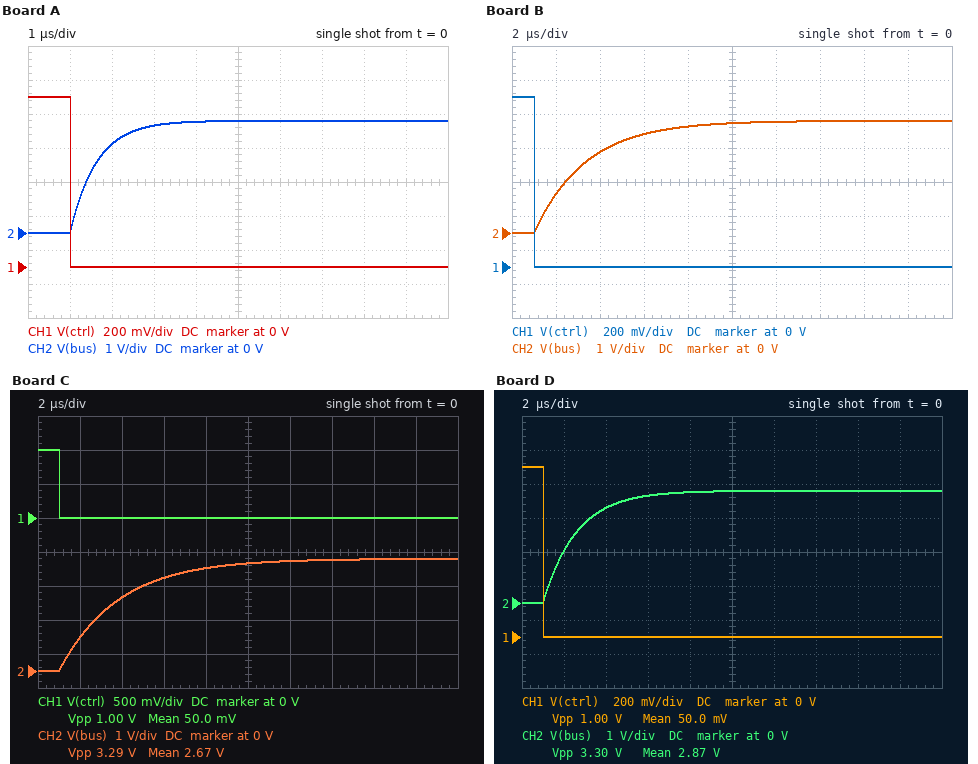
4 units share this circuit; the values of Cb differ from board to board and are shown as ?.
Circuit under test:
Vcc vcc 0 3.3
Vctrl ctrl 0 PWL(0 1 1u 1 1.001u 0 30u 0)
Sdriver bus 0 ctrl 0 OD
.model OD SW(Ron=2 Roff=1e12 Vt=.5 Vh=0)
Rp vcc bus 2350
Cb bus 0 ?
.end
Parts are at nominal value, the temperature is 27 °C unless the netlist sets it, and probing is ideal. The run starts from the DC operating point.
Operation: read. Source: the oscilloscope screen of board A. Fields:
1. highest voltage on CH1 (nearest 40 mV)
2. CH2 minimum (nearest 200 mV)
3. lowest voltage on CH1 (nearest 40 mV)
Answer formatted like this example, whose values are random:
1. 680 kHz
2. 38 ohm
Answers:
1. 1.00 V
2. 0 V
3. 0 V
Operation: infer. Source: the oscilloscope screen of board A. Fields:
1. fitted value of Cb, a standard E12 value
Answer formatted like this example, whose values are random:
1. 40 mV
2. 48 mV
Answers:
1. 270 pF
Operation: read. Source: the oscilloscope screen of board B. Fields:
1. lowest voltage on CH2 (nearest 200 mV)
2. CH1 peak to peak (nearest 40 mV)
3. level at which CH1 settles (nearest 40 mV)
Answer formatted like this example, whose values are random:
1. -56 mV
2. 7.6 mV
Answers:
1. 0 V
2. 1.00 V
3. 0 V
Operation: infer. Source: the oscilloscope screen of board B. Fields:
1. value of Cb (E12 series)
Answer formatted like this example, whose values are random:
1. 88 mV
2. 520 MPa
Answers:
1. 1 nF
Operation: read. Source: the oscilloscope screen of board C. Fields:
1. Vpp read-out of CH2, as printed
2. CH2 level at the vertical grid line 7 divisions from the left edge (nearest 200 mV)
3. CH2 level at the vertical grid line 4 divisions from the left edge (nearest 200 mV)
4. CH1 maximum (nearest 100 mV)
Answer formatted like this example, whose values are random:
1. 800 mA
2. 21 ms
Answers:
1. 3.29 V
2. 3.2 V
3. 3.0 V
4. 1.0 V
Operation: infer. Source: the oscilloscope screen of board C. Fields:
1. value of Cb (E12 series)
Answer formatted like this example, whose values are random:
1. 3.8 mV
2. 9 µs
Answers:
1. 1.2 nF
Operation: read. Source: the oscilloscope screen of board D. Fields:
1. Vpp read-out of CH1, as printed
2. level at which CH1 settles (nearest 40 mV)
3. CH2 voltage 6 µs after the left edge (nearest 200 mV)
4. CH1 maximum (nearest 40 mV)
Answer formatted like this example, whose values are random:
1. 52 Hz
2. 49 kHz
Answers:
1. 1.00 V
2. 0 V
3. 3.2 V
4. 1.00 V
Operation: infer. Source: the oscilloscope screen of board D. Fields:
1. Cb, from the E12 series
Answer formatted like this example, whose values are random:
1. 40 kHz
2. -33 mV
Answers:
1. 680 pF
